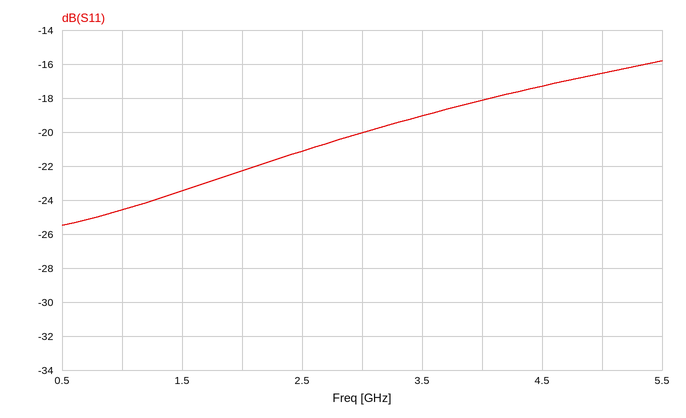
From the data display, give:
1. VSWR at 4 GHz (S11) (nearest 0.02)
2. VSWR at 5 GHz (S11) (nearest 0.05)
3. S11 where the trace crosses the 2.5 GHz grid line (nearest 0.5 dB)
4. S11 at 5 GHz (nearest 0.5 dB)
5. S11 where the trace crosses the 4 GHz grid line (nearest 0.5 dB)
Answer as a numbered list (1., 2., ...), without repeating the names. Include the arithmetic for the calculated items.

1. |Γ| = 10^(-18/20) = 0.1259; VSWR = (1 + 0.1259)/(1 − 0.1259) ≈ 1.29, so 1.28 to the nearest 0.02
2. |Γ| = 10^(-16.5/20) = 0.1496; VSWR = (1 + 0.1496)/(1 − 0.1496) ≈ 1.35
3. -21.0 dB
4. -16.5 dB
5. -18.0 dB
